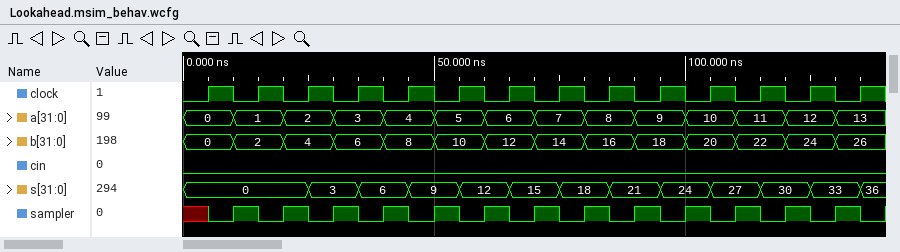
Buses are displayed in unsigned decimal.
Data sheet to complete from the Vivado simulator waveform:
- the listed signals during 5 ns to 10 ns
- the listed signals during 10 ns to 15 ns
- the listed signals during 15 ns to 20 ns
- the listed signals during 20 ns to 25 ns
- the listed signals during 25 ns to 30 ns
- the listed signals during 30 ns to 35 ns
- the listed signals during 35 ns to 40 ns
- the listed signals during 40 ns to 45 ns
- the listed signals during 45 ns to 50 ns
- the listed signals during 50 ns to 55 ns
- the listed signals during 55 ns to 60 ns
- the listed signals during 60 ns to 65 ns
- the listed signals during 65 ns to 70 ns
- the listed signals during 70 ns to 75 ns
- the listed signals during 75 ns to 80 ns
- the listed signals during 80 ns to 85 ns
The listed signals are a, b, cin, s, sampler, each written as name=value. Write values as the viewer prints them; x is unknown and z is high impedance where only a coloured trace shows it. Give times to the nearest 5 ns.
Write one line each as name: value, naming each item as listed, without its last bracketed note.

the listed signals during 5 ns to 10 ns: a=0, b=0, cin=0, s=0, sampler=0
the listed signals during 10 ns to 15 ns: a=1, b=2, cin=0, s=0, sampler=1
the listed signals during 15 ns to 20 ns: a=1, b=2, cin=0, s=0, sampler=0
the listed signals during 20 ns to 25 ns: a=2, b=4, cin=0, s=0, sampler=1
the listed signals during 25 ns to 30 ns: a=2, b=4, cin=0, s=3, sampler=0
the listed signals during 30 ns to 35 ns: a=3, b=6, cin=0, s=3, sampler=1
the listed signals during 35 ns to 40 ns: a=3, b=6, cin=0, s=6, sampler=0
the listed signals during 40 ns to 45 ns: a=4, b=8, cin=0, s=6, sampler=1
the listed signals during 45 ns to 50 ns: a=4, b=8, cin=0, s=9, sampler=0
the listed signals during 50 ns to 55 ns: a=5, b=10, cin=0, s=9, sampler=1
the listed signals during 55 ns to 60 ns: a=5, b=10, cin=0, s=12, sampler=0
the listed signals during 60 ns to 65 ns: a=6, b=12, cin=0, s=12, sampler=1
the listed signals during 65 ns to 70 ns: a=6, b=12, cin=0, s=15, sampler=0
the listed signals during 70 ns to 75 ns: a=7, b=14, cin=0, s=15, sampler=1
the listed signals during 75 ns to 80 ns: a=7, b=14, cin=0, s=18, sampler=0
the listed signals during 80 ns to 85 ns: a=8, b=16, cin=0, s=18, sampler=1
